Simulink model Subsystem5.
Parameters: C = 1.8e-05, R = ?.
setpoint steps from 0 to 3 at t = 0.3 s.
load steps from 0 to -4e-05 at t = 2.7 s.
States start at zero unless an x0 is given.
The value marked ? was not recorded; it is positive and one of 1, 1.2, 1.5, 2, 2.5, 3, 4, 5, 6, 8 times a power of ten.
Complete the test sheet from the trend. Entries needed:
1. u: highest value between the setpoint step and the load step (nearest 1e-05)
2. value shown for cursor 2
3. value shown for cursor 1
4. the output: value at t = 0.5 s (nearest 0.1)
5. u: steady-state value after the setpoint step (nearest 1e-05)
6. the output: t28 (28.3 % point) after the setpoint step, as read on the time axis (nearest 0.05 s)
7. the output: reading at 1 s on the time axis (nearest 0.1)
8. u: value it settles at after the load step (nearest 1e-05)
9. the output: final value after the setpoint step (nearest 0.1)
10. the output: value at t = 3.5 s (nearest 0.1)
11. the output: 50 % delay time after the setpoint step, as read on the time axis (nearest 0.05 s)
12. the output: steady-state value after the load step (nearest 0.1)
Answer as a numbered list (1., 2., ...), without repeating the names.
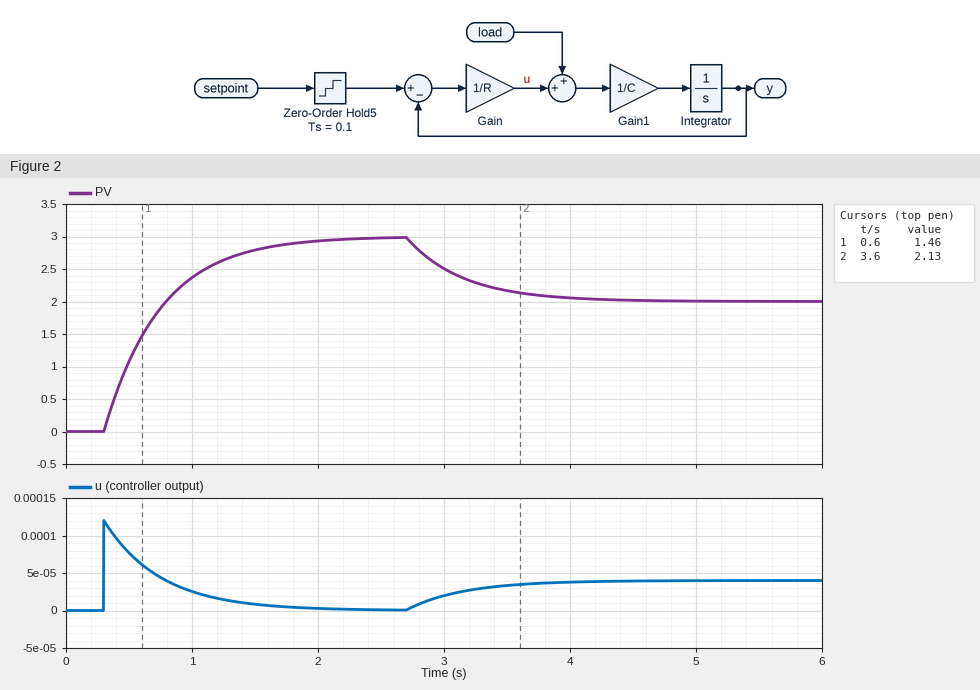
1. 0.00012
2. 2.13
3. 1.46
4. 1.1
5. 0.00000
6. 0.45 s
7. 2.4
8. 0.00004
9. 3.0
10. 2.2
11. 0.60 s
12. 2.0
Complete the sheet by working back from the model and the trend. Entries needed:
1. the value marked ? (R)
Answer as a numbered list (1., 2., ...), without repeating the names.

1. 25000
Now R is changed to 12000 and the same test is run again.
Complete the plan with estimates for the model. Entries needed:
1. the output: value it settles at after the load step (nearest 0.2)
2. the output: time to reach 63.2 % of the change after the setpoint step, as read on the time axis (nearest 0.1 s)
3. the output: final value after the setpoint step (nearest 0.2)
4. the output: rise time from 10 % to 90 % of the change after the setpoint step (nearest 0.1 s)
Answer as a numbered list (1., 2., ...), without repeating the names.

1. 2.6
2. 0.5 s
3. 3.0
4. 0.5 s
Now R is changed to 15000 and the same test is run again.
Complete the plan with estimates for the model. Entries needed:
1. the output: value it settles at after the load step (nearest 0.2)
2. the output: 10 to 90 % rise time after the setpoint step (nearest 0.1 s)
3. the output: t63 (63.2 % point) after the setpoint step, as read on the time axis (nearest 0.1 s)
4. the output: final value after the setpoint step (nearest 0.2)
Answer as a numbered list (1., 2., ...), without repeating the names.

1. 2.4
2. 0.6 s
3. 0.6 s
4. 3.0
